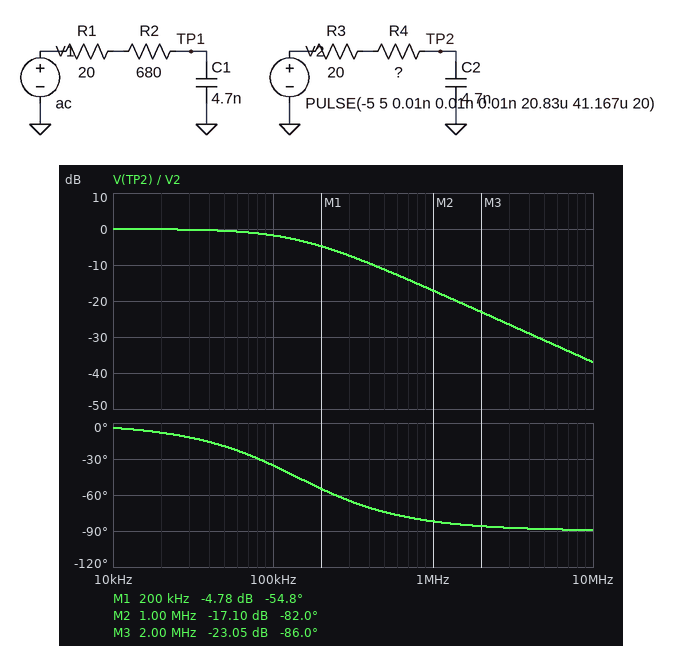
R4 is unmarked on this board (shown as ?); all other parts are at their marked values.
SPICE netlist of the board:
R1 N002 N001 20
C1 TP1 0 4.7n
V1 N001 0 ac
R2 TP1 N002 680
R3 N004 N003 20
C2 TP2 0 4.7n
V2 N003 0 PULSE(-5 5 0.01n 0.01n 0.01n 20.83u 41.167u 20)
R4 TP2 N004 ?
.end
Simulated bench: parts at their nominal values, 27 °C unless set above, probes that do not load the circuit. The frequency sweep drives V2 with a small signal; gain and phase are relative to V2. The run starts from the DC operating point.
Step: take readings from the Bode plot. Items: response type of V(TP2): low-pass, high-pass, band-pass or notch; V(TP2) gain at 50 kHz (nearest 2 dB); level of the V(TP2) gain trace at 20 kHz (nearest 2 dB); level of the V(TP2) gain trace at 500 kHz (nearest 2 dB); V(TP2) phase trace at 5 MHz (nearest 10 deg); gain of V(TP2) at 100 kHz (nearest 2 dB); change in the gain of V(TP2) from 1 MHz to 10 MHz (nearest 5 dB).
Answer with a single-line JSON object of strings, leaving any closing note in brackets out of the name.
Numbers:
{"response type of V(TP2): low-pass, high-pass, band-pass or notch": "low-pass", "V(TP2) gain at 50 kHz": "0 dB", "level of the V(TP2) gain trace at 20 kHz": "0 dB", "level of the V(TP2) gain trace at 500 kHz": "-12 dB", "V(TP2) phase trace at 5 MHz": "-90 deg", "gain of V(TP2) at 100 kHz": "-2 dB", "change in the gain of V(TP2) from 1 MHz to 10 MHz": "-20 dB"}
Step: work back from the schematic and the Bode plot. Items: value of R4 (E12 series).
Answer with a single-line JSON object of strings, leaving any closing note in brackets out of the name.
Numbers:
{"value of R4": "220 Ω"}
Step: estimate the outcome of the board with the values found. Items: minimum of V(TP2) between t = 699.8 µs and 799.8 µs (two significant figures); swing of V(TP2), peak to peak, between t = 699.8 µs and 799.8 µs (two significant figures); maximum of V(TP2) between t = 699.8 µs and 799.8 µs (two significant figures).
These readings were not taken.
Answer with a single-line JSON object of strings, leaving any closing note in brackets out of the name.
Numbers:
{"minimum of V(TP2) between t = 699.8 µs and 799.8 µs": "-5.0 V", "swing of V(TP2), peak to peak, between t = 699.8 µs and 799.8 µs": "10 V", "maximum of V(TP2) between t = 699.8 µs and 799.8 µs": "5.0 V"}
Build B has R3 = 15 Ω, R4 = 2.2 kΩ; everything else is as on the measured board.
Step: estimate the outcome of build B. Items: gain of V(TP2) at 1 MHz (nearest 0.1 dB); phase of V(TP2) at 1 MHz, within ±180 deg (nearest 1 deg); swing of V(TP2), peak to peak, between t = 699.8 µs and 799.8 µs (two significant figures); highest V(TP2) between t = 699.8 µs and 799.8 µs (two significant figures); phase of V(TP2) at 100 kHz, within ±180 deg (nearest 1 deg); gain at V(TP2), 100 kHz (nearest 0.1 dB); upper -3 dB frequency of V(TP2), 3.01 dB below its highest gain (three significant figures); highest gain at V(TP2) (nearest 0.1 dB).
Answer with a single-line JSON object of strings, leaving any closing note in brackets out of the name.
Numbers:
{"gain of V(TP2) at 1 MHz": "-36.3 dB", "phase of V(TP2) at 1 MHz, within ±180 deg": "-89 deg", "swing of V(TP2), peak to peak, between t = 699.8 µs and 799.8 µs": "7.6 V", "highest V(TP2) between t = 699.8 µs and 799.8 µs": "3.8 V", "phase of V(TP2) at 100 kHz, within ±180 deg": "-81 deg", "gain at V(TP2), 100 kHz": "-16.4 dB", "upper -3 dB frequency of V(TP2), 3.01 dB below its highest gain": "15.3 kHz", "highest gain at V(TP2)": "0 dB"}
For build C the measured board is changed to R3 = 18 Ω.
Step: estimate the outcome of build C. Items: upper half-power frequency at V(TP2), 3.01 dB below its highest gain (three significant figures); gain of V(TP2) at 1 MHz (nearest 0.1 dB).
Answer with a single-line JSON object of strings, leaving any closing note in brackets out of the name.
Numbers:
{"upper half-power frequency at V(TP2), 3.01 dB below its highest gain": "142 kHz", "gain of V(TP2) at 1 MHz": "-17.0 dB"}
